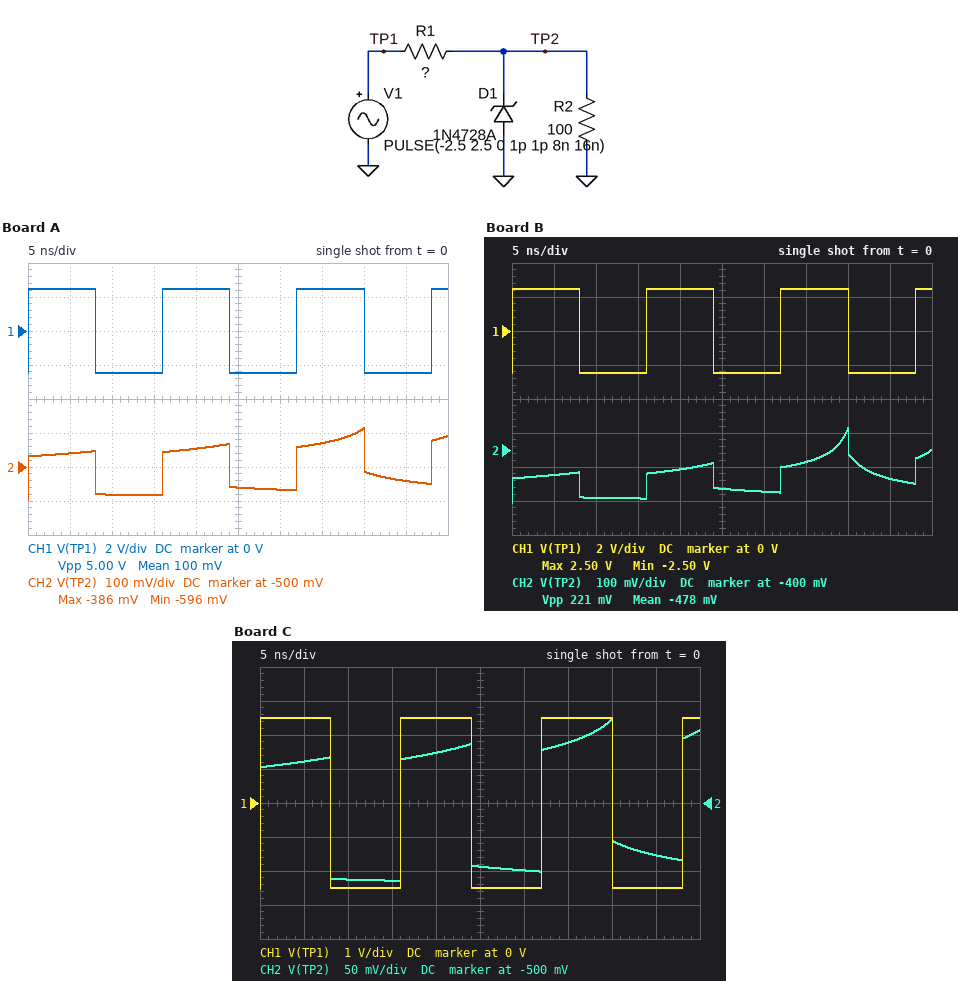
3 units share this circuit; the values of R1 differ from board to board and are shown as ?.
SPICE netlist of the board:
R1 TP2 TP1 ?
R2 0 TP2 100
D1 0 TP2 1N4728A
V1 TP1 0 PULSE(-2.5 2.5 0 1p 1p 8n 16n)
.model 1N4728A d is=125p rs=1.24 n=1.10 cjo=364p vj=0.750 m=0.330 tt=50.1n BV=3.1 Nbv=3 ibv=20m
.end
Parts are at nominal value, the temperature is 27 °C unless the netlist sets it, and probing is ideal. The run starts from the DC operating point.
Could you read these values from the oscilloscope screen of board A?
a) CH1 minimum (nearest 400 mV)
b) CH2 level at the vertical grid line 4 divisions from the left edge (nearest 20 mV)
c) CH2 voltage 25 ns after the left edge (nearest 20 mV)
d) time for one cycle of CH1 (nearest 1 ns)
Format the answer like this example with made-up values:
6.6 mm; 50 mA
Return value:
-2.4 V; -440 mV; -560 mV; 16 ns
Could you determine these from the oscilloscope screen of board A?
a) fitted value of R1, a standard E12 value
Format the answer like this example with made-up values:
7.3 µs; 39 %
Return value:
47 Ω
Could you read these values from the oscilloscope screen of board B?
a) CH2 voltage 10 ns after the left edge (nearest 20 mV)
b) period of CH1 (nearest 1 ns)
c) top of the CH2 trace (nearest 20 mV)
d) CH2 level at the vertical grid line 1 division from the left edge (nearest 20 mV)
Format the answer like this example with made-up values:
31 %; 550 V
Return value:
-540 mV; 16 ns; -340 mV; -480 mV
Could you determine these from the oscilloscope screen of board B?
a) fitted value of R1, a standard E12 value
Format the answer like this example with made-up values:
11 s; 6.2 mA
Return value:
82 Ω
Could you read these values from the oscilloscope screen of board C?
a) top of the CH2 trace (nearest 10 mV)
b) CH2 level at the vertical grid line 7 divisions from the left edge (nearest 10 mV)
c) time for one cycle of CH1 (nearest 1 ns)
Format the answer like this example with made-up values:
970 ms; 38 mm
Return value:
-380 mV; -410 mV; 16 ns
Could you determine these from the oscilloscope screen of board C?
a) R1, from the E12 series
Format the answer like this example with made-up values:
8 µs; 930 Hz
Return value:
33 Ω
